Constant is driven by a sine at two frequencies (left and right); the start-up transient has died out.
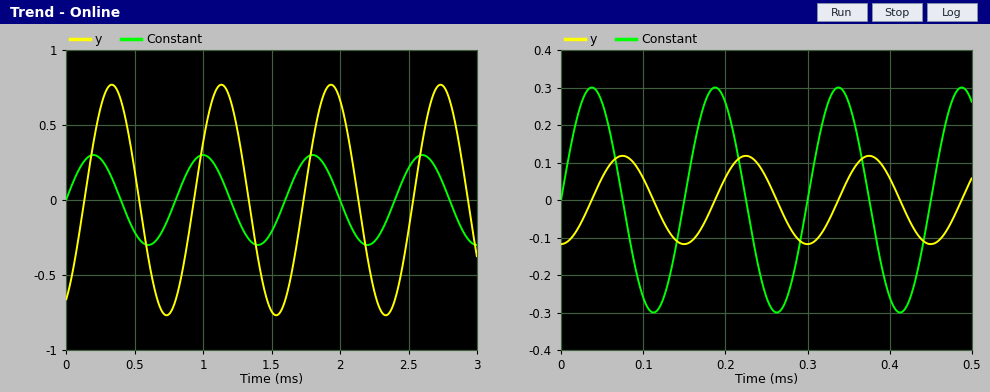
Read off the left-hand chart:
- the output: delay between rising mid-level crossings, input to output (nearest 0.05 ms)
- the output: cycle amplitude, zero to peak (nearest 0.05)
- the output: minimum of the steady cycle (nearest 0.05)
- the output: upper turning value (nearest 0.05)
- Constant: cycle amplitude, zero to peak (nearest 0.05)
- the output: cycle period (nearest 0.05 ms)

0.15 ms
0.75
-0.75
0.75
0.30
0.80 ms
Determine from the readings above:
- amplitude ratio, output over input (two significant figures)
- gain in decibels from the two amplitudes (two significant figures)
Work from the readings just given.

2.5
8.0 dB
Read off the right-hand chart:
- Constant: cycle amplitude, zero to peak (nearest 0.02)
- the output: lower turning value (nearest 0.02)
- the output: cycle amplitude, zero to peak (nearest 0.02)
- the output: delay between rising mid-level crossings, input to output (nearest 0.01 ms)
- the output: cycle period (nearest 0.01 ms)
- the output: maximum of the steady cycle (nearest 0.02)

0.30
-0.12
0.12
0.04 ms
0.15 ms
0.12
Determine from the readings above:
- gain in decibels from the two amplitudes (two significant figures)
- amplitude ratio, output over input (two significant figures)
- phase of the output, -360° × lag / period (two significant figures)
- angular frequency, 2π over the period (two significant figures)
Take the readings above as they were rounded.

-8.0 dB
0.40
-96°
42 rad/ms
